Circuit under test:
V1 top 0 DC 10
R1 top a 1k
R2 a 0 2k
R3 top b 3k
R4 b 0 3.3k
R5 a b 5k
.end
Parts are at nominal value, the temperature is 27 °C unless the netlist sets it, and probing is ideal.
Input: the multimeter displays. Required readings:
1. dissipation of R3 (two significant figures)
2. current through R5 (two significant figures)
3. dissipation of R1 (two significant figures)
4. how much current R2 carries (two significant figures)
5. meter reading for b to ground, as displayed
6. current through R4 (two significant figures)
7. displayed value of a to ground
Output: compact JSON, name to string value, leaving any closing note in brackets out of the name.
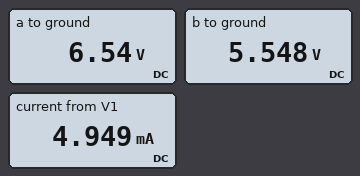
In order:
{"dissipation of R3": "6.6 mW", "current through R5": "200 µA", "dissipation of R1": "12 mW", "how much current R2 carries": "3.3 mA", "meter reading for b to ground, as displayed": "5.548 V", "current through R4": "1.7 mA", "displayed value of a to ground": "6.54 V"}
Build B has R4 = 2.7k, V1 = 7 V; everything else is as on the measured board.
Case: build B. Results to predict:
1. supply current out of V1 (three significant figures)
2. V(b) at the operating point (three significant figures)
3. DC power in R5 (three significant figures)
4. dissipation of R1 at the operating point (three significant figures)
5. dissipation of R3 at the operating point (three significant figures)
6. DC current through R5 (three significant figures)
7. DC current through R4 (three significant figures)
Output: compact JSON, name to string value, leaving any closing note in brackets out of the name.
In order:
{"supply current out of V1": "3.60 mA", "V(b) at the operating point": "3.59 V", "DC power in R5": "182 µW", "dissipation of R1 at the operating point": "6.05 mW", "dissipation of R3 at the operating point": "3.88 mW", "DC current through R5": "191 µA", "DC current through R4": "1.33 mA"}
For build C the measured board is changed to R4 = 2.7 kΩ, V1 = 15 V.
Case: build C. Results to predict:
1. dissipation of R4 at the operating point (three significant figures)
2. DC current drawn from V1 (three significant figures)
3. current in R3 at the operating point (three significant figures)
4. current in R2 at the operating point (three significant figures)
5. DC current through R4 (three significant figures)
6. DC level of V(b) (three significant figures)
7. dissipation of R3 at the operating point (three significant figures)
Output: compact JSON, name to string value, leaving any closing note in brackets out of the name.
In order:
{"dissipation of R4 at the operating point": "21.9 mW", "DC current drawn from V1": "7.71 mA", "current in R3 at the operating point": "2.44 mA", "current in R2 at the operating point": "4.86 mA", "DC current through R4": "2.85 mA", "DC level of V(b)": "7.69 V", "dissipation of R3 at the operating point": "17.8 mW"}
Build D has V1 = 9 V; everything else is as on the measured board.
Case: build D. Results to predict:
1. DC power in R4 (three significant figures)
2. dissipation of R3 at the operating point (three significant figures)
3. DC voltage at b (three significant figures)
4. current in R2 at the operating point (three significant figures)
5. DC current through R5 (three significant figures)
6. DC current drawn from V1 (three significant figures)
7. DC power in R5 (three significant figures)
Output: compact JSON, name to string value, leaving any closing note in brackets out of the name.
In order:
{"DC power in R4": "7.56 mW", "dissipation of R3 at the operating point": "5.35 mW", "DC voltage at b": "4.99 V", "current in R2 at the operating point": "2.94 mA", "DC current through R5": "178 µA", "DC current drawn from V1": "4.45 mA", "DC power in R5": "158 µW"}
